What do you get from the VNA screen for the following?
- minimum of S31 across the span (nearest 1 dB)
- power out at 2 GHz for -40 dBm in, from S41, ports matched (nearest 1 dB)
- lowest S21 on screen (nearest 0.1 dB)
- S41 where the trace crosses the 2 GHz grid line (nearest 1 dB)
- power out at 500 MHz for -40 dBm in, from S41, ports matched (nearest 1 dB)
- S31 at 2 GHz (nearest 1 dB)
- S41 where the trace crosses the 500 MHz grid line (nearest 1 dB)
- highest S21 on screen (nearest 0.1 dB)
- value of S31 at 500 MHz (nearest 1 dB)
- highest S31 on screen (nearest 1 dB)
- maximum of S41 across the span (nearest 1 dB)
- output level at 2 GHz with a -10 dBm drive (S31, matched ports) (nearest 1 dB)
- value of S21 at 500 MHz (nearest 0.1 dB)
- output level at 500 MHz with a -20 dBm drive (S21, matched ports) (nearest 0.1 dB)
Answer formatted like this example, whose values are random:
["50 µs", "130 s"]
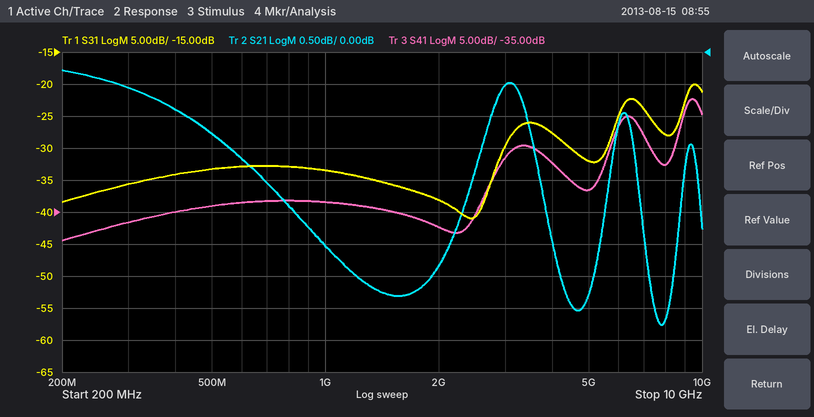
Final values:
["-41 dB", "-77 dBm", "-4.3 dB", "-37 dB", "-74 dBm", "-38 dB", "-34 dB", "-0.3 dB", "-33 dB", "-20 dB", "-17 dB", "-48 dBm", "-1.3 dB", "-21.3 dBm"]
